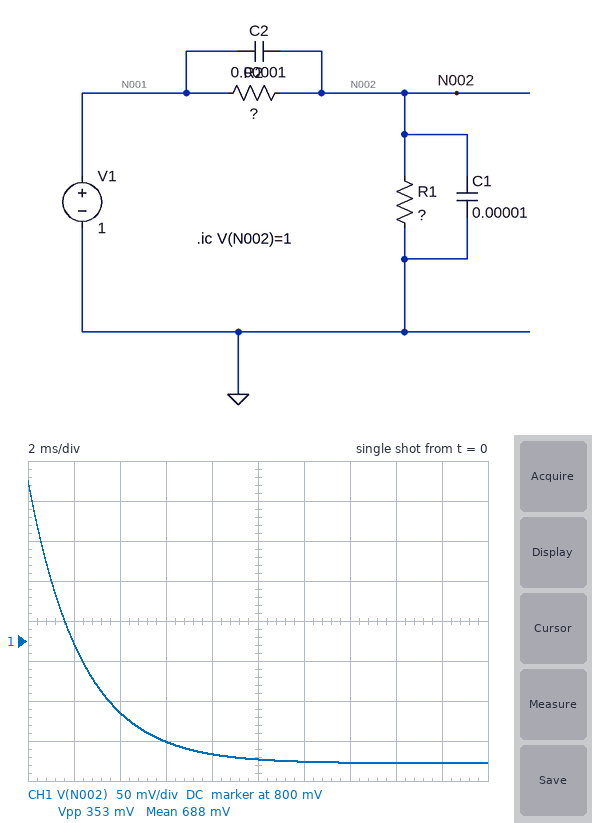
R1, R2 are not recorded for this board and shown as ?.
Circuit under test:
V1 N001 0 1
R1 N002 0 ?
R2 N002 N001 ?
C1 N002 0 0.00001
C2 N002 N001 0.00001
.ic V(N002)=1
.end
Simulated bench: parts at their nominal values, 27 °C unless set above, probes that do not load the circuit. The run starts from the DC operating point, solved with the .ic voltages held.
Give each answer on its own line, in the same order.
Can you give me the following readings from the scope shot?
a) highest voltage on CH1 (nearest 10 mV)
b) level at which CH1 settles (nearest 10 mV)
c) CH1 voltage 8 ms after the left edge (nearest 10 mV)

1.00 V
650 mV
660 mV
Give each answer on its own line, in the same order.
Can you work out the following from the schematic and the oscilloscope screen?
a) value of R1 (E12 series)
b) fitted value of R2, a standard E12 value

330 Ω
180 Ω
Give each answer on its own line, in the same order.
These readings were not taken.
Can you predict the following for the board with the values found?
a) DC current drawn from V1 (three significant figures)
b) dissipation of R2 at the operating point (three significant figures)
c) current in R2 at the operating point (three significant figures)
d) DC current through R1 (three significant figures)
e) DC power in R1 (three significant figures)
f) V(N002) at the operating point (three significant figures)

1.96 mA
692 µW
1.96 mA
1.96 mA
1.27 mW
647 mV
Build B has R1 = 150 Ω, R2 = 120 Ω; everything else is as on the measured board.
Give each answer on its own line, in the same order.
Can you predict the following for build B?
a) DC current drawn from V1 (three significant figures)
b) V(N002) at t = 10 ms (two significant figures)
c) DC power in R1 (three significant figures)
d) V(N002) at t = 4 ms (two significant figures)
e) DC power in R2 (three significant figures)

3.70 mA
560 mV
2.06 mW
580 mV
1.65 mW
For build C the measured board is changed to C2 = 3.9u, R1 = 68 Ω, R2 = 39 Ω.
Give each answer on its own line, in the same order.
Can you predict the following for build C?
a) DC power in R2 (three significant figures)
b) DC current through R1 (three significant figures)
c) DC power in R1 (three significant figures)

3.41 mW
9.35 mA
5.94 mW
